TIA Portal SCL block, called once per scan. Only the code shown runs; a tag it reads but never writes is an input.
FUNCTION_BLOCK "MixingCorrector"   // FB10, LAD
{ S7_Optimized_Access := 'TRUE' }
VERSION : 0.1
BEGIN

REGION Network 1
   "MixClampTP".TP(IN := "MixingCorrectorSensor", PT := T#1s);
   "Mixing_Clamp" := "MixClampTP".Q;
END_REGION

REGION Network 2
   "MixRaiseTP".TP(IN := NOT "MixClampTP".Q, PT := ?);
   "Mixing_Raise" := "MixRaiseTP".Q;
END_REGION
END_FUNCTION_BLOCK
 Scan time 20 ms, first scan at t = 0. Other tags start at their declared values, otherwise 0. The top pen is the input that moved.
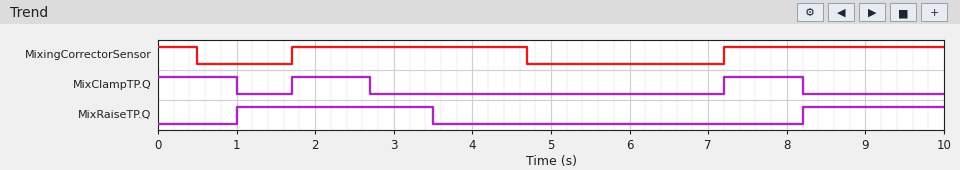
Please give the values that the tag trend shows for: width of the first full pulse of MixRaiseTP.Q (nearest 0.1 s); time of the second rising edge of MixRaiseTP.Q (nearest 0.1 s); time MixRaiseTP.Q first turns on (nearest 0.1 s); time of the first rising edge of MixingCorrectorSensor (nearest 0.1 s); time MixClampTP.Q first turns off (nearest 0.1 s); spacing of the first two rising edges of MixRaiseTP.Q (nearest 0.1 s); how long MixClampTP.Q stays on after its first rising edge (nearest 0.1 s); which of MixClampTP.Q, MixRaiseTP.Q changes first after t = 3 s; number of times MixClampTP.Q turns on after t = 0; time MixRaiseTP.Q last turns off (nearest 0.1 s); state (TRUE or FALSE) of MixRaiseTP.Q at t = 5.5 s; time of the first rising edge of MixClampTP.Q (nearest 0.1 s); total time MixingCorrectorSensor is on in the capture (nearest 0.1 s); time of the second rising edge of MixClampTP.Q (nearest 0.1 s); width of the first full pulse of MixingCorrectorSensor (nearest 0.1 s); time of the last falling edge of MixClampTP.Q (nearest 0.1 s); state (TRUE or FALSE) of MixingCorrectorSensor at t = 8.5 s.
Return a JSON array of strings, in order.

["2.5 s", "8.2 s", "1.0 s", "1.7 s", "1.0 s", "7.2 s", "1.0 s", "MixRaiseTP.Q", "2", "3.5 s", "FALSE", "1.7 s", "6.3 s", "7.2 s", "3.0 s", "8.2 s", "TRUE"]
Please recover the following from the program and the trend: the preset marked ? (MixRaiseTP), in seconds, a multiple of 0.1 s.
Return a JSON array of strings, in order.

["2.5 s"]
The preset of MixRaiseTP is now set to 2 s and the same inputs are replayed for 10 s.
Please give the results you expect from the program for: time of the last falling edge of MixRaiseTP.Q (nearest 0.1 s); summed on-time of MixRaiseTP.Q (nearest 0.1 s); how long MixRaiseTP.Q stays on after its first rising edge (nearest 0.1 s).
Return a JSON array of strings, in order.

["3.0 s", "3.8 s", "2.0 s"]
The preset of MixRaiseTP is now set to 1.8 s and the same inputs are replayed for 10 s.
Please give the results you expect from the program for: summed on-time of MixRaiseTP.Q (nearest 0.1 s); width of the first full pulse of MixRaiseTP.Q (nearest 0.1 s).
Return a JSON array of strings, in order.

["3.6 s", "1.8 s"]
